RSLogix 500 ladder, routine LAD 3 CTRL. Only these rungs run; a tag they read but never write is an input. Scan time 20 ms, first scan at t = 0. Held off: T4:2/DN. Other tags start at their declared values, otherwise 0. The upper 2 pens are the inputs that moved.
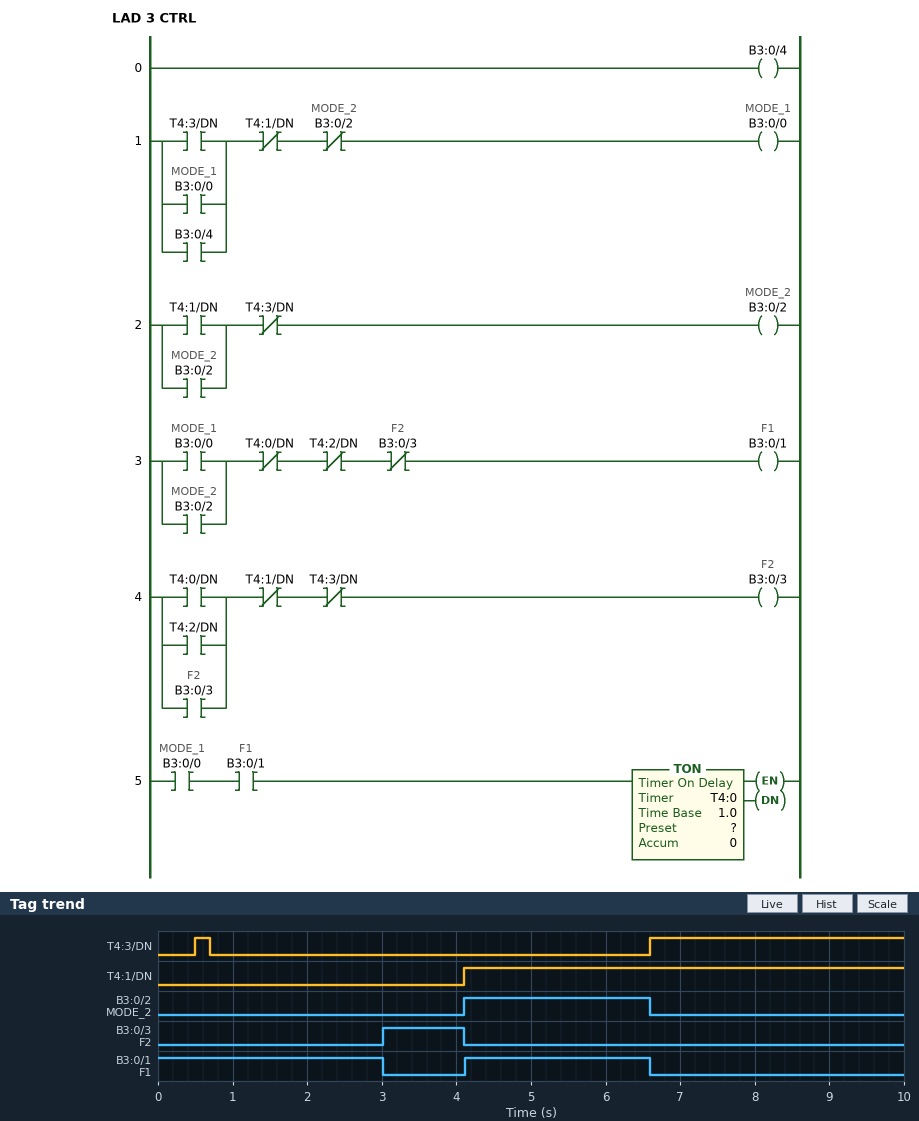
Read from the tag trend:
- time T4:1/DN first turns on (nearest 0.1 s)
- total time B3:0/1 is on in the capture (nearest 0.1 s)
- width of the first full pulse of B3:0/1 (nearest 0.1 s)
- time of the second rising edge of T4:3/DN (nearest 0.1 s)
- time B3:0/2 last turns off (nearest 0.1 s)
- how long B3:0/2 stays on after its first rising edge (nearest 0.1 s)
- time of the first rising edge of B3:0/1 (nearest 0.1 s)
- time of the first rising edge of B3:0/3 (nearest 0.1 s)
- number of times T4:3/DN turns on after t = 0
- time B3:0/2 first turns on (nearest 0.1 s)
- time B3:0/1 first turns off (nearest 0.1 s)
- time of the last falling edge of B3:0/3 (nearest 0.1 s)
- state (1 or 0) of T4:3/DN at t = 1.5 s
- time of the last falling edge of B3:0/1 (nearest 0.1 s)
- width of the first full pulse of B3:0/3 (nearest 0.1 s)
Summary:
4.1 s
5.5 s
2.5 s
6.6 s
6.6 s
2.5 s
4.1 s
3.0 s
2
4.1 s
3.0 s
4.1 s
0
6.6 s
1.1 s
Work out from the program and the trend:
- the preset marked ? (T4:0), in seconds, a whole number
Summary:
3 s
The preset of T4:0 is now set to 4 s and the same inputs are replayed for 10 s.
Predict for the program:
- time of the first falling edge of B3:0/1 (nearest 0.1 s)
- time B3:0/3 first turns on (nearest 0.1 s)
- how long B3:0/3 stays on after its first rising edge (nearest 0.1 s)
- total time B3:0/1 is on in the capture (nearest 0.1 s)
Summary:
4.0 s
4.0 s
0.1 s
6.5 s
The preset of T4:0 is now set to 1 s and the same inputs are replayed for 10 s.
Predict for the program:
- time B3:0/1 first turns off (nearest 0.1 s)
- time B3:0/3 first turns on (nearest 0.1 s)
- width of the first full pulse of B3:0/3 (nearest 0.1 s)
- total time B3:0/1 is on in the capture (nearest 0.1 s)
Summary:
1.0 s
1.0 s
3.1 s
3.5 s
